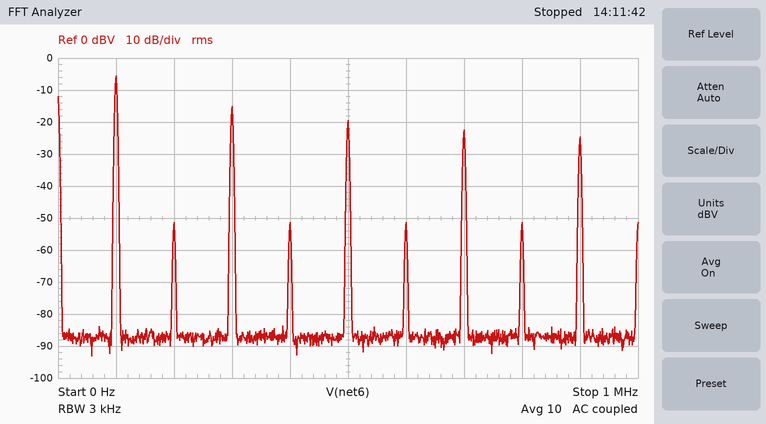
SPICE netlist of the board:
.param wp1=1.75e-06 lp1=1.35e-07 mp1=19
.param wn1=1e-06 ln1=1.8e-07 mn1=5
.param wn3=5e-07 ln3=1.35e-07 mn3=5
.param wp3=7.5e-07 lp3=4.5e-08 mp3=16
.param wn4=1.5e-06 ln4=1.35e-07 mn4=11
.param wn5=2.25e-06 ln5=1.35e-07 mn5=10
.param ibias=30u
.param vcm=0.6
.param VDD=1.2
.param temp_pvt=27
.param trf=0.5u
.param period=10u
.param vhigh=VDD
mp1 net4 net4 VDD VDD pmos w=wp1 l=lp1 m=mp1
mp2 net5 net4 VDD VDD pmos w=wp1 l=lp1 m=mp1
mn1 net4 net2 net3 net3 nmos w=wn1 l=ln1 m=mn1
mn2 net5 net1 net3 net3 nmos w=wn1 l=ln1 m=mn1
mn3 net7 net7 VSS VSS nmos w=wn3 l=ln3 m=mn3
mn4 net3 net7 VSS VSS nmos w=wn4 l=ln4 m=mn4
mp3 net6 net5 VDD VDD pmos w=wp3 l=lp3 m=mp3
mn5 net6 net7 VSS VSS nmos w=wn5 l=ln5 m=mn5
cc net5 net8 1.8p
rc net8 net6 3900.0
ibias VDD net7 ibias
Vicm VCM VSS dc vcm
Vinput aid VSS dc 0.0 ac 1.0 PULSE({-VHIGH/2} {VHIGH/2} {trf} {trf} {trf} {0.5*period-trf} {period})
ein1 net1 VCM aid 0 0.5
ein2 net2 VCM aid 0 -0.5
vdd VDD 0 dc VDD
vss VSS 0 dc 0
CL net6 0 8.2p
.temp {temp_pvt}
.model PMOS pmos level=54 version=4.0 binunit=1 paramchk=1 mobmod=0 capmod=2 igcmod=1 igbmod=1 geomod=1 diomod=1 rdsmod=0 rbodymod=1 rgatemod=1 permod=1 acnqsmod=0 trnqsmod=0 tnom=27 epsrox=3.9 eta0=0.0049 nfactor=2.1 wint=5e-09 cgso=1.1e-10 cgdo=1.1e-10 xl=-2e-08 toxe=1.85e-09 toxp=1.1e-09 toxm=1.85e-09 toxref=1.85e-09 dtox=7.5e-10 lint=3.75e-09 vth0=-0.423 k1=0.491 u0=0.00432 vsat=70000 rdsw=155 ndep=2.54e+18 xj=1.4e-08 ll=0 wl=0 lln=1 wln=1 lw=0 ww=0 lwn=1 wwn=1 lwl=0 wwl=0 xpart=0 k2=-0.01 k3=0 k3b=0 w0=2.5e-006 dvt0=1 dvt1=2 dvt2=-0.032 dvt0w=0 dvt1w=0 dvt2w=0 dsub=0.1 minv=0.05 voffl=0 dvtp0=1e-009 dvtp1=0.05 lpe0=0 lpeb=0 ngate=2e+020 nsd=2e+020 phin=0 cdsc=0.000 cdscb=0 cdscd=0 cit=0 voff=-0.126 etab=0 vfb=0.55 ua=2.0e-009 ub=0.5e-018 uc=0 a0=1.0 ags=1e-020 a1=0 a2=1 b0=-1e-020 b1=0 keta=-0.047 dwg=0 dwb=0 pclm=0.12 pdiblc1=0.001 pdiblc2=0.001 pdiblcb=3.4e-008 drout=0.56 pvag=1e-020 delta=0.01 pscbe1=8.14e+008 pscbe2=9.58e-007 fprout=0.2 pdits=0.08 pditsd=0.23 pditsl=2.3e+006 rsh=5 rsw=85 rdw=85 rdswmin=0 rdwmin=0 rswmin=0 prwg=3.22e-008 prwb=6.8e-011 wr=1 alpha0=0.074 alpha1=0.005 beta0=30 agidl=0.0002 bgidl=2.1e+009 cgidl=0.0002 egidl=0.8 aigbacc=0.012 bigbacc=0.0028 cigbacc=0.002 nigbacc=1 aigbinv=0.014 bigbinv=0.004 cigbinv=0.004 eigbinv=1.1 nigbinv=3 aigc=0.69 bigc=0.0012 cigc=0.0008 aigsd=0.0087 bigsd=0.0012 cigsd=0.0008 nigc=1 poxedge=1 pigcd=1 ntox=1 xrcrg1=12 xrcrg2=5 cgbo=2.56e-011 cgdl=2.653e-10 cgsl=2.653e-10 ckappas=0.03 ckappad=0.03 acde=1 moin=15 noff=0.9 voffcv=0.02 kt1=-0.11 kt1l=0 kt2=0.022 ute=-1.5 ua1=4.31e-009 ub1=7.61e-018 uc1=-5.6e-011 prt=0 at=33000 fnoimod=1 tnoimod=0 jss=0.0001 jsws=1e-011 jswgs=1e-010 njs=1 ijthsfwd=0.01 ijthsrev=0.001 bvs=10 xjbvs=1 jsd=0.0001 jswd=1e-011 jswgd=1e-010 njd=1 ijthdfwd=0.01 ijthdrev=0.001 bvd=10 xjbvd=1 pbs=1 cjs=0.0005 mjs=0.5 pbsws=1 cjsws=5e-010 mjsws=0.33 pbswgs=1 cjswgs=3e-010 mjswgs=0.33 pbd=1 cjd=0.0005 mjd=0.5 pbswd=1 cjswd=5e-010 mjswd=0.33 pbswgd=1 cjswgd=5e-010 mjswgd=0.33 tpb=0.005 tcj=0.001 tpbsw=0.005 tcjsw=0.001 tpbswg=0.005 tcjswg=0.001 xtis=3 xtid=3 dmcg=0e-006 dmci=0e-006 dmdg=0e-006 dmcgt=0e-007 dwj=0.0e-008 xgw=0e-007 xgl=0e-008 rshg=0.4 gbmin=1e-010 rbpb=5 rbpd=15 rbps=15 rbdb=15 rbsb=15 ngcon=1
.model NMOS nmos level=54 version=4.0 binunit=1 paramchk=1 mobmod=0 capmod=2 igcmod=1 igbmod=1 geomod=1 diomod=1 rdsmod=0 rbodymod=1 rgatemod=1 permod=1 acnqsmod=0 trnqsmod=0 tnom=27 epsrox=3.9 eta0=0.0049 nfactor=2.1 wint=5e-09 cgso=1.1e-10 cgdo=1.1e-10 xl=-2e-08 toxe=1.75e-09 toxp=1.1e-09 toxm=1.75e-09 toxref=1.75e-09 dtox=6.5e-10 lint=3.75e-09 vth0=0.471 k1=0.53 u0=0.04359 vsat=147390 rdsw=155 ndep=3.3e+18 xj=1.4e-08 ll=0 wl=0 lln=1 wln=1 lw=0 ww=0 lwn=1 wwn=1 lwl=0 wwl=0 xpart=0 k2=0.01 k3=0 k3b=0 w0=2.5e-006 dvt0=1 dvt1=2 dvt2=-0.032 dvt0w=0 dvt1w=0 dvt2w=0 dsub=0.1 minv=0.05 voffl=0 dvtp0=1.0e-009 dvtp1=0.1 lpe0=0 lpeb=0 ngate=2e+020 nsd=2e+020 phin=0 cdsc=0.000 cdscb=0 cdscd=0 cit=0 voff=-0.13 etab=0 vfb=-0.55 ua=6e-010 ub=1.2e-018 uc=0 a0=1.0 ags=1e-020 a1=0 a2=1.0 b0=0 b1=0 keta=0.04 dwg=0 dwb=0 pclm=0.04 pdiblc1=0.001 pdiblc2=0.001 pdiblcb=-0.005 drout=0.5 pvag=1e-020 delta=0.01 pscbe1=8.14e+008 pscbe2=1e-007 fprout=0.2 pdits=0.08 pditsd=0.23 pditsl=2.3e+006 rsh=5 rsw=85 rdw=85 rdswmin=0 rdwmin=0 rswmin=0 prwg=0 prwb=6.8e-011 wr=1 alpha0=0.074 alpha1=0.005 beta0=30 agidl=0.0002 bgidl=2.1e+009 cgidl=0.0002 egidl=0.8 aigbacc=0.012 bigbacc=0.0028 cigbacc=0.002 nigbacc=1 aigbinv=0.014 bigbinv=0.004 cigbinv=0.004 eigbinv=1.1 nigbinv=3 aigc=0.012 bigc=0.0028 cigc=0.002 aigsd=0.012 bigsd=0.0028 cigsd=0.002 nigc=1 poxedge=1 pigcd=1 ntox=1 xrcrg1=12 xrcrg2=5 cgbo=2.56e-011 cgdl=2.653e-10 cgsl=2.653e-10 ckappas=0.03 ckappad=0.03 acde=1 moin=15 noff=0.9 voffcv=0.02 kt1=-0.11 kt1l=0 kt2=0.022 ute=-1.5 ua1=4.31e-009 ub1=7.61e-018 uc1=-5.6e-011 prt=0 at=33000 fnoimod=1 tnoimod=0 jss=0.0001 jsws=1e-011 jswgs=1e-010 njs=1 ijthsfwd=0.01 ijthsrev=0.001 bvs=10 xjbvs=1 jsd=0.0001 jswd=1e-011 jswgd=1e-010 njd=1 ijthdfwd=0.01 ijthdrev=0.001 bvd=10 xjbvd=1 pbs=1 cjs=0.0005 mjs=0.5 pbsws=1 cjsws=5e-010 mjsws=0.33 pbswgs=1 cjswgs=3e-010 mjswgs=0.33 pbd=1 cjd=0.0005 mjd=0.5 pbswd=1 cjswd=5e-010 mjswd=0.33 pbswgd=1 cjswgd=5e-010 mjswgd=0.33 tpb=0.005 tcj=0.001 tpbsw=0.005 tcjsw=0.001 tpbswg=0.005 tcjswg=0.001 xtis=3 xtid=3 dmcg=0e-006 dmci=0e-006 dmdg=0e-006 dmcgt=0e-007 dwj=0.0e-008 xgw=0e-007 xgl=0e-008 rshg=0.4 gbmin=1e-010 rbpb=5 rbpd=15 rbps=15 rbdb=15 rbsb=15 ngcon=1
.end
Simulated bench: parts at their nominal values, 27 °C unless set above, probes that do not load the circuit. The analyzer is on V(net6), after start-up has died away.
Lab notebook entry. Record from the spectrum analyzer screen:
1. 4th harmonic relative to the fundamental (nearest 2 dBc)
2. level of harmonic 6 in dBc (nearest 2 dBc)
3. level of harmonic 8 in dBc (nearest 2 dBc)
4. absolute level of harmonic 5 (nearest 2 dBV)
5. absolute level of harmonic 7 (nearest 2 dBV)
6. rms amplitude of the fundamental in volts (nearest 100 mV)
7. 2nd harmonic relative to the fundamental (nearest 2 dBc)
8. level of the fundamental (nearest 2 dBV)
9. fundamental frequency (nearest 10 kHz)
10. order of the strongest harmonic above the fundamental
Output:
-46 dBc
-46 dBc
-46 dBc
-20 dBV
-22 dBV
500 mV
-46 dBc
-6 dBV
100 kHz
3
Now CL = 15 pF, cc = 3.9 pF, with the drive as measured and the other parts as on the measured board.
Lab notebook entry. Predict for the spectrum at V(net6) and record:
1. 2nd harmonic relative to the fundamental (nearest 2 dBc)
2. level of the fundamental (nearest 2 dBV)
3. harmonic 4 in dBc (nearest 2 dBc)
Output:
-40 dBc
-6 dBV
-40 dBc
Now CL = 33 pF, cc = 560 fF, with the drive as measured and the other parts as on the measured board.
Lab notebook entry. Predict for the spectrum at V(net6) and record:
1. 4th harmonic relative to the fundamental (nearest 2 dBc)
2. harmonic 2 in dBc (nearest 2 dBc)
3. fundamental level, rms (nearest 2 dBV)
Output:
-34 dBc
-34 dBc
-6 dBV
